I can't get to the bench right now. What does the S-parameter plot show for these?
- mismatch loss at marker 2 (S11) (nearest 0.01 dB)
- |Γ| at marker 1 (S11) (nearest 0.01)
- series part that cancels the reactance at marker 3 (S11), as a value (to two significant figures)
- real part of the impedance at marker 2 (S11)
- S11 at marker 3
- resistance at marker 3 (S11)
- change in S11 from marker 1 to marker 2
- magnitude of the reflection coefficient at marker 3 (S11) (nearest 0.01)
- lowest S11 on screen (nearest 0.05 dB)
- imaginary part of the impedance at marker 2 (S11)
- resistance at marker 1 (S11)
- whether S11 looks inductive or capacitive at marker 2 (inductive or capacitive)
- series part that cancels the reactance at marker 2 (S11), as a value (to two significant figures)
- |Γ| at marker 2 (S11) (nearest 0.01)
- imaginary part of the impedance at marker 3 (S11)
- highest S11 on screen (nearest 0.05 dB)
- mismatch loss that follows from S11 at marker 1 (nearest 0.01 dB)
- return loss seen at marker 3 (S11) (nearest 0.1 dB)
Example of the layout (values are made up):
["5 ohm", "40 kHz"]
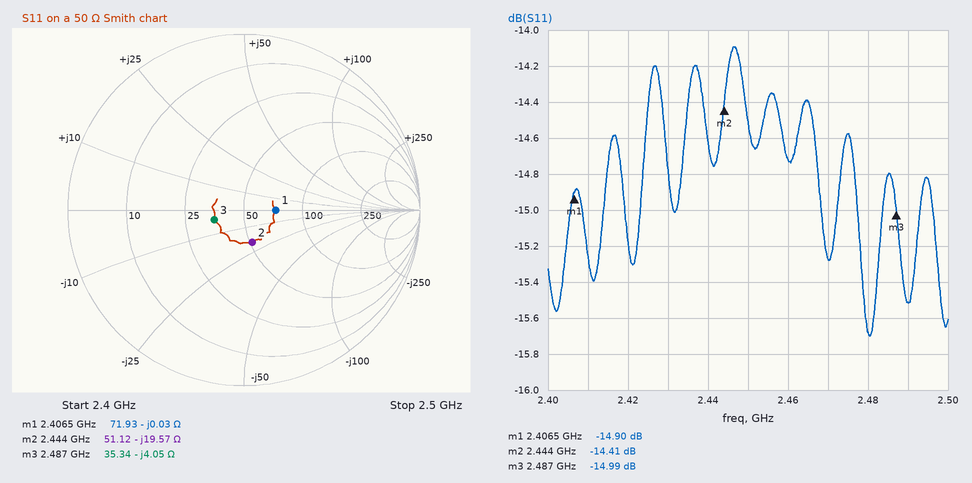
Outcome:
["0.16 dB", "0.18", "260 pH", "51.12 Ω", "-14.99 dB", "35.34 Ω", "0.49 dB", "0.18", "-15.70 dB", "-19.57 Ω", "71.93 Ω", "capacitive", "1.3 nH", "0.19", "-4.05 Ω", "-14.10 dB", "0.14 dB", "15.0 dB"]
